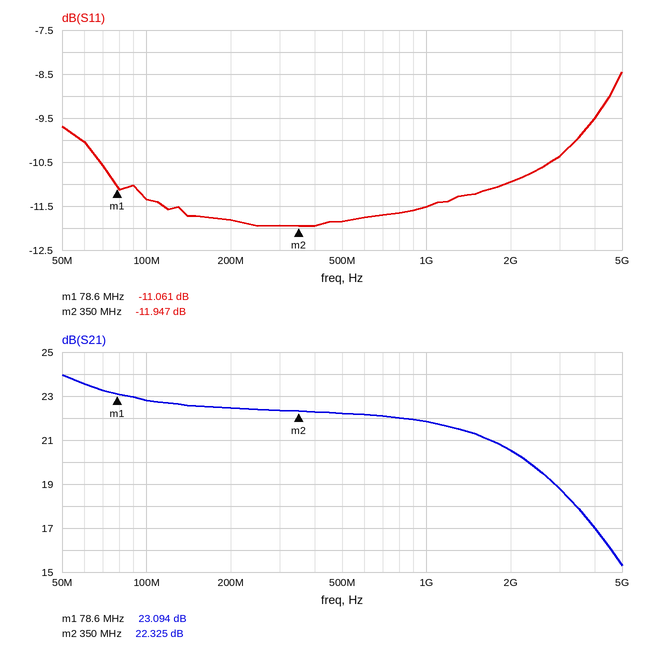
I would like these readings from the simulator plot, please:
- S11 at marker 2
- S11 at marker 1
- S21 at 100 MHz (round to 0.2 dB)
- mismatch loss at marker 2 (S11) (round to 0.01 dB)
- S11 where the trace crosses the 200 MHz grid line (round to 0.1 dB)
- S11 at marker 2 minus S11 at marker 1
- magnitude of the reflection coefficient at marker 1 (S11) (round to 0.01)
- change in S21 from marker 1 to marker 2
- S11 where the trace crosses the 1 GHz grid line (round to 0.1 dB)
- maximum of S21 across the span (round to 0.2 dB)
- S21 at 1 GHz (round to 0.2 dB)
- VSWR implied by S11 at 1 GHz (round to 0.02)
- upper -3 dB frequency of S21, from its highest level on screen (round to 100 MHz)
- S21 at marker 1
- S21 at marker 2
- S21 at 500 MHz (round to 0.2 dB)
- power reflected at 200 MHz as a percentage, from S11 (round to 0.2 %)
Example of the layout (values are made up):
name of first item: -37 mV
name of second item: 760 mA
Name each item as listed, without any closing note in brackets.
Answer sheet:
S11 at marker 2: -11.947 dB
S11 at marker 1: -11.061 dB
S21 at 100 MHz: 22.8 dB
mismatch loss at marker 2 (S11): 0.29 dB
S11 where the trace crosses the 200 MHz grid line: -11.8 dB
S11 at marker 2 minus S11 at marker 1: -0.886 dB
magnitude of the reflection coefficient at marker 1 (S11): 0.28
change in S21 from marker 1 to marker 2: -0.769 dB
S11 where the trace crosses the 1 GHz grid line: -11.5 dB
maximum of S21 across the span: 24.0 dB
S21 at 1 GHz: 21.8 dB
VSWR implied by S11 at 1 GHz: 1.72
upper -3 dB frequency of S21, from its highest level on screen: 1.7 GHz
S21 at marker 1: 23.094 dB
S21 at marker 2: 22.325 dB
S21 at 500 MHz: 22.2 dB
power reflected at 200 MHz as a percentage, from S11: 6.6 %
